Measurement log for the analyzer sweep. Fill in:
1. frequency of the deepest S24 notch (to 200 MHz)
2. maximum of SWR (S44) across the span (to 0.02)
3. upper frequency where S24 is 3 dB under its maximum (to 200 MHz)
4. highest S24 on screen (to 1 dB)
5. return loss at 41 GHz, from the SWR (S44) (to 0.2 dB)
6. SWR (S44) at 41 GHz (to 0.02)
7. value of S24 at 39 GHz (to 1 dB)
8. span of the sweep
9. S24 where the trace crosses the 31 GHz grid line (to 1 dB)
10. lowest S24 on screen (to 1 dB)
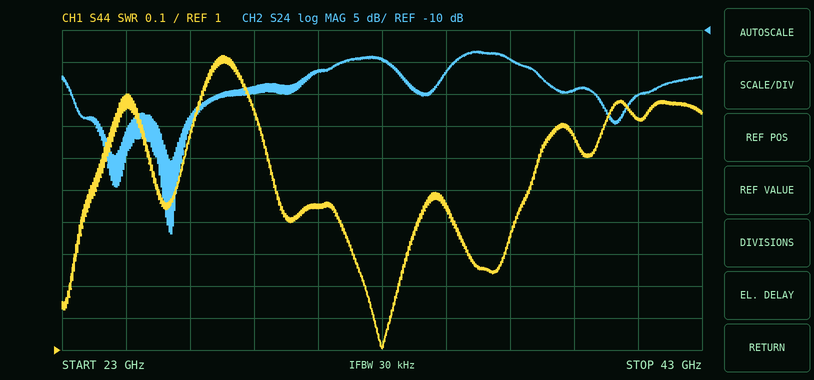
26.4 GHz
1.92
37.8 GHz
-13 dB
11.6 dB
1.72
-19 dB
20 GHz
-16 dB
-42 dB
